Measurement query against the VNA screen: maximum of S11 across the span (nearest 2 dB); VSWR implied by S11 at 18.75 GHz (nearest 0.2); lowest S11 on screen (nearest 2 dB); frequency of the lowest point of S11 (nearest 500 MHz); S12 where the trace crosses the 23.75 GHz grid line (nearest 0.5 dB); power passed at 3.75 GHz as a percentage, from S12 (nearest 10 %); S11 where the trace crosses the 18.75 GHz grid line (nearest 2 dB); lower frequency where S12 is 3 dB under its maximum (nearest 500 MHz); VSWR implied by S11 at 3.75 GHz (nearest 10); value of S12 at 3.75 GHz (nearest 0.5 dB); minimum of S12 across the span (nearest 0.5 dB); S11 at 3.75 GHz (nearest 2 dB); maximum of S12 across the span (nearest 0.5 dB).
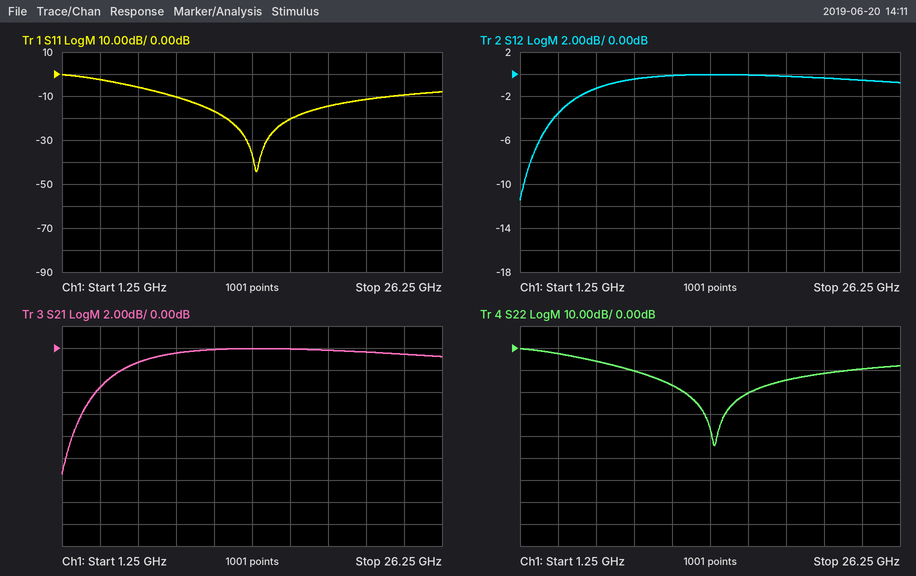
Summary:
0 dB
1.4
-44 dB
14.0 GHz
-0.5 dB
40 %
-14 dB
4.0 GHz
10
-3.5 dB
-11.5 dB
-2 dB
0.0 dB
